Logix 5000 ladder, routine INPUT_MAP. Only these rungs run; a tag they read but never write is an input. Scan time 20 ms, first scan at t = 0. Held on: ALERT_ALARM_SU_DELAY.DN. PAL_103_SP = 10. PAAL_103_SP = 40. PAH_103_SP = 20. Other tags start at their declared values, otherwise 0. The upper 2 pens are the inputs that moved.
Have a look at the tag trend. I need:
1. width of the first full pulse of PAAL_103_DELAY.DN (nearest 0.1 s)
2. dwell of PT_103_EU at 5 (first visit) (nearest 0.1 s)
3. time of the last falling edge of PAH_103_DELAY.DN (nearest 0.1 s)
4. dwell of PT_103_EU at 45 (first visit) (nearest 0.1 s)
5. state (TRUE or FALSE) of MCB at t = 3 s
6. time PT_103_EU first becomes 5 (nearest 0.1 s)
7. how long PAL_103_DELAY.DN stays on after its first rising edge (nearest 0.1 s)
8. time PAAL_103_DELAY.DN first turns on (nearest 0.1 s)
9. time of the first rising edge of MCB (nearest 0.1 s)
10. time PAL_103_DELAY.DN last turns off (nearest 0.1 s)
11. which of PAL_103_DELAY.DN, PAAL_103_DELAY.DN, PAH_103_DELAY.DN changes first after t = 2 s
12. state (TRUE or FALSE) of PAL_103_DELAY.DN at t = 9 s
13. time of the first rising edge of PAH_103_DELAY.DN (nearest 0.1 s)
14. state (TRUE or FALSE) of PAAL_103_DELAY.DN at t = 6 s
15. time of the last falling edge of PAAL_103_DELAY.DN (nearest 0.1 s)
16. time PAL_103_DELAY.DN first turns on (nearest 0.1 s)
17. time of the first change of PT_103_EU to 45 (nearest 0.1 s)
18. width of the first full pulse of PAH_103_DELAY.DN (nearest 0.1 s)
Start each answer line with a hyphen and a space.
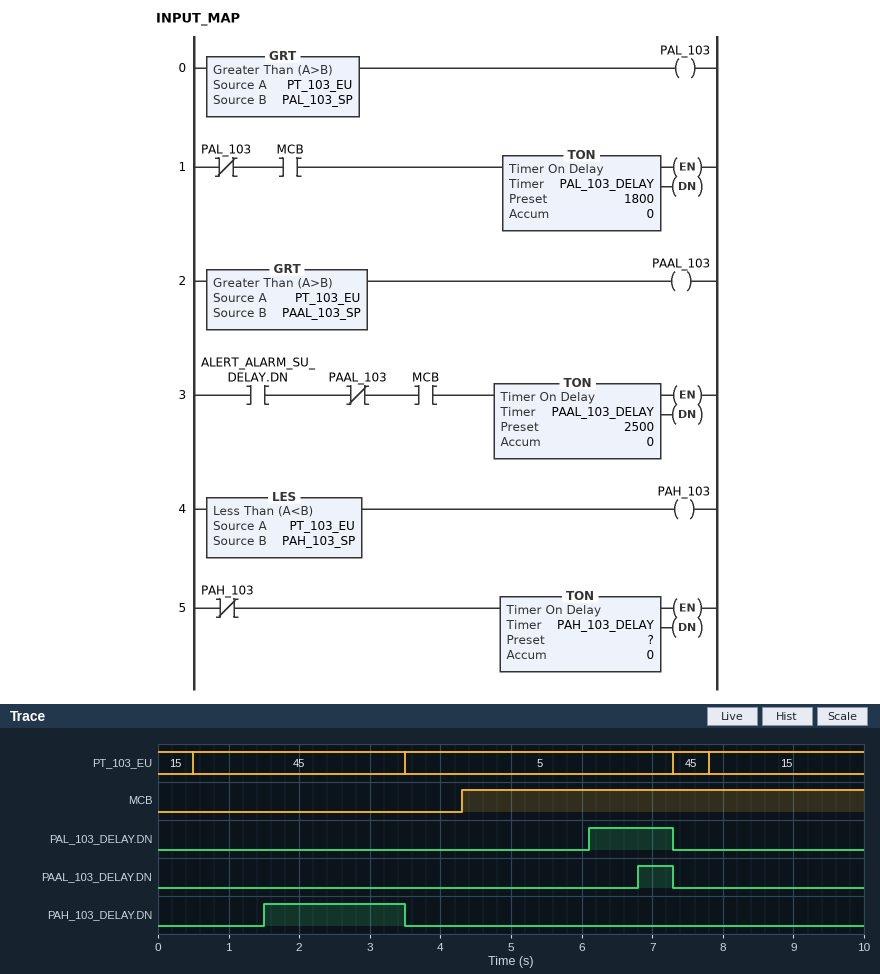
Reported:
- 0.5 s
- 3.8 s
- 3.5 s
- 3.0 s
- FALSE
- 3.5 s
- 1.2 s
- 6.8 s
- 4.3 s
- 7.3 s
- PAH_103_DELAY.DN
- FALSE
- 1.5 s
- FALSE
- 7.3 s
- 6.1 s
- 0.5 s
- 2.0 s
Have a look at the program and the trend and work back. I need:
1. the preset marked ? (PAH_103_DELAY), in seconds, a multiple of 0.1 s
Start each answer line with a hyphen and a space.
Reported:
- 1.0 s
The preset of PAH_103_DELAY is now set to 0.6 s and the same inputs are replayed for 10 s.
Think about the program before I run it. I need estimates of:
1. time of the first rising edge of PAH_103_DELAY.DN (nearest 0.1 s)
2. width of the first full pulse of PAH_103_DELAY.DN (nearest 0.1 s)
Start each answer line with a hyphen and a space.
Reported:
- 1.1 s
- 2.4 s
